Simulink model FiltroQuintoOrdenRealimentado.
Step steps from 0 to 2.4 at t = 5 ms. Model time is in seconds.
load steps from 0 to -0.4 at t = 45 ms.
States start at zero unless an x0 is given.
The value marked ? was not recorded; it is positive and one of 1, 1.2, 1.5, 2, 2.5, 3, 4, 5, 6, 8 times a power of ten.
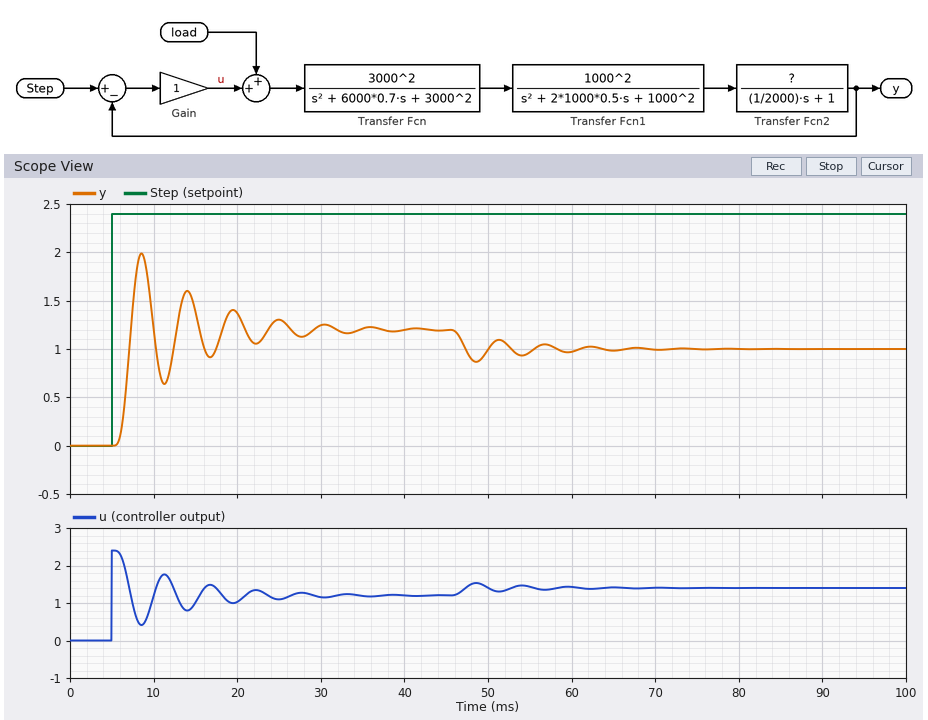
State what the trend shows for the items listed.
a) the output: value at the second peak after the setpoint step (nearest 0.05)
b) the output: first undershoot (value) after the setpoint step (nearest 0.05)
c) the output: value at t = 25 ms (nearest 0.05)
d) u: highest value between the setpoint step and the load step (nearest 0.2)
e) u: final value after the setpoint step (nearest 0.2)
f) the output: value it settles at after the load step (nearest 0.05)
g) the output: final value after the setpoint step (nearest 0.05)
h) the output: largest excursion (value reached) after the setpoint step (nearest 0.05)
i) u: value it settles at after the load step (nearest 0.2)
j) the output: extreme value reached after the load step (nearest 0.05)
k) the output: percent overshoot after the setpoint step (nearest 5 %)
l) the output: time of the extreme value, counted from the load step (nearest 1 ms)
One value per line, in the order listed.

1.60
0.65
1.30
2.4
1.2
1.00
1.20
2.00
1.4
0.85
65 %
4 ms
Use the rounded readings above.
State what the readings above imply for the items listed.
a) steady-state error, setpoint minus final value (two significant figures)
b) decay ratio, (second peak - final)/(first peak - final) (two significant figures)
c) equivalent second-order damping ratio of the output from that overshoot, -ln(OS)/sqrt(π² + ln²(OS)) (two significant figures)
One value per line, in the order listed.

1.2
0.50
0.14
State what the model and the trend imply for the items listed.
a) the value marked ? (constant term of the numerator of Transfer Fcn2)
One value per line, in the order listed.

1
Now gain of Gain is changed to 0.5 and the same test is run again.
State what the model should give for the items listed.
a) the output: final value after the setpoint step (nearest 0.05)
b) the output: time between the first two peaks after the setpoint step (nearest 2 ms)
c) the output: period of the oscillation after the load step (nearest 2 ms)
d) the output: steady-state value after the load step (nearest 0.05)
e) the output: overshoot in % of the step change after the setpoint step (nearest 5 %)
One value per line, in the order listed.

0.80
6 ms
6 ms
0.55
40 %
